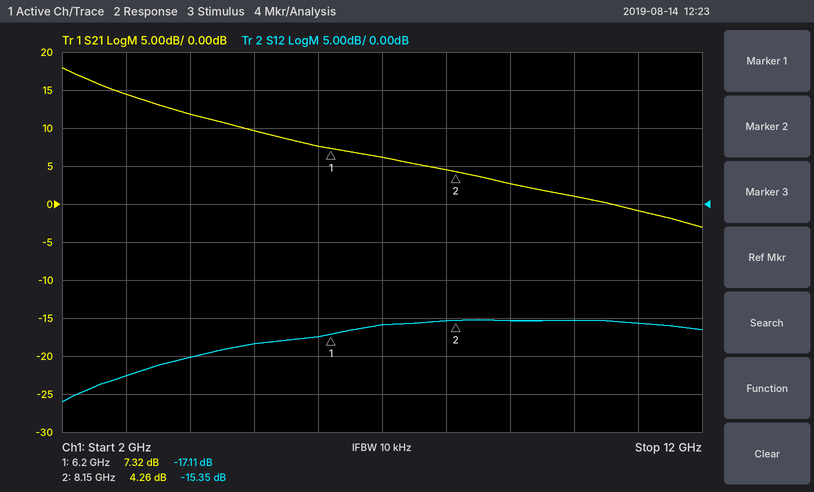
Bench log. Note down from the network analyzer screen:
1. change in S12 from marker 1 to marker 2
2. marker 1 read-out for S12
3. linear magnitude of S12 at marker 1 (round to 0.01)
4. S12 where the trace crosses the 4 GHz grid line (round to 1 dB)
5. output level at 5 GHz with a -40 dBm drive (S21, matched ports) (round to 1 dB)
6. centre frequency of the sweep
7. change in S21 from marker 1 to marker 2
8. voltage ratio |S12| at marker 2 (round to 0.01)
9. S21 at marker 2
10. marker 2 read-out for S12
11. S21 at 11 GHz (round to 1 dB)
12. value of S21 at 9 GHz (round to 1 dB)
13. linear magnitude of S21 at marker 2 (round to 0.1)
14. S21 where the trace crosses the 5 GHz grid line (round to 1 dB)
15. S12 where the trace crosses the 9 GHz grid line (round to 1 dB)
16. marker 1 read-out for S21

1.76 dB
-17.11 dB
0.14
-20 dB
-30 dBm
7 GHz
-3.06 dB
0.17
4.26 dB
-15.35 dB
-1 dB
3 dB
1.6
10 dB
-15 dB
7.32 dB
